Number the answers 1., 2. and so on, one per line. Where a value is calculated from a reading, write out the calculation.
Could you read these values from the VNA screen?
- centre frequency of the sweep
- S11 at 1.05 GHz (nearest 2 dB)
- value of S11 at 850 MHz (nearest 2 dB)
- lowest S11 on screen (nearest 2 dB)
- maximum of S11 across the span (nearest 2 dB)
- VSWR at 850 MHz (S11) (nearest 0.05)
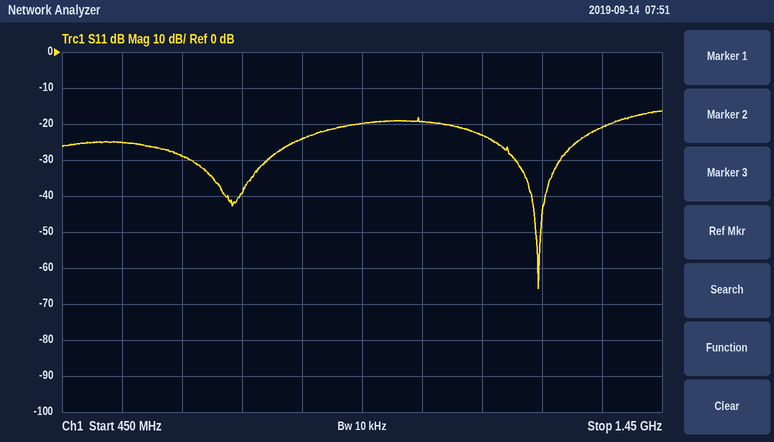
1. 950 MHz
2. -20 dB
3. -24 dB
4. -66 dB
5. -16 dB
6. |Γ| = 10^(-24/20) = 0.0631; VSWR = (1 + 0.0631)/(1 − 0.0631) ≈ 1.13, so 1.15 to the nearest 0.05
